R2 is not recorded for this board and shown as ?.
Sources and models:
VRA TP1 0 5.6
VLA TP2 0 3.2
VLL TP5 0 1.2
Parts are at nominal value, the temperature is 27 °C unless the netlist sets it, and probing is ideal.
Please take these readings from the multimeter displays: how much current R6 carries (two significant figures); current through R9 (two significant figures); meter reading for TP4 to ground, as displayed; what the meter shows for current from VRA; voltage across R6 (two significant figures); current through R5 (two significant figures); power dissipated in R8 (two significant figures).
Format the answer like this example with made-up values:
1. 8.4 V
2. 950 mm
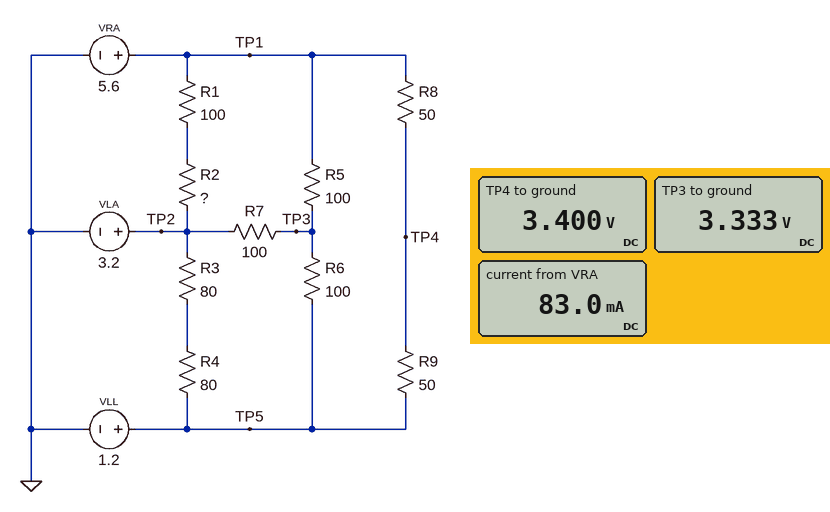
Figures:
1. 21 mA
2. 44 mA
3. 3.400 V
4. 83.0 mA
5. 2.1 V
6. 23 mA
7. 97 mW
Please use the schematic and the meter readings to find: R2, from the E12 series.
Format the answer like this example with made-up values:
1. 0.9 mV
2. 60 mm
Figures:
1. 47 Ω
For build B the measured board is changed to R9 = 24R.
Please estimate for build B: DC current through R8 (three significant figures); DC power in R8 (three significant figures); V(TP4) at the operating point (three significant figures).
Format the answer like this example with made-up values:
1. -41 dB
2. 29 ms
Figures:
1. 59.5 mA
2. 177 mW
3. 2.63 V
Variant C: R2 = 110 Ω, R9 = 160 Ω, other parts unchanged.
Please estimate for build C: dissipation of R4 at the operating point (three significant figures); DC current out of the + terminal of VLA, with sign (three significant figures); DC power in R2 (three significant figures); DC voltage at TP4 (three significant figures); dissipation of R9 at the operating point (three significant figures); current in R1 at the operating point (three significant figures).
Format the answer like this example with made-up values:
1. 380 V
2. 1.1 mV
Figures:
1. 12.5 mW
2. -262 µA
3. 14.4 mW
4. 4.55 V
5. 70.2 mW
6. 11.4 mA
